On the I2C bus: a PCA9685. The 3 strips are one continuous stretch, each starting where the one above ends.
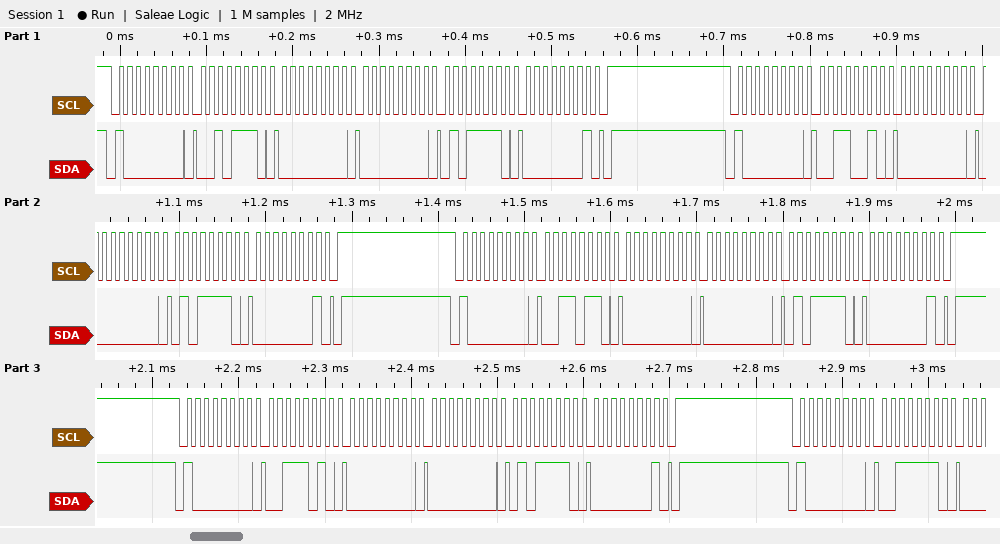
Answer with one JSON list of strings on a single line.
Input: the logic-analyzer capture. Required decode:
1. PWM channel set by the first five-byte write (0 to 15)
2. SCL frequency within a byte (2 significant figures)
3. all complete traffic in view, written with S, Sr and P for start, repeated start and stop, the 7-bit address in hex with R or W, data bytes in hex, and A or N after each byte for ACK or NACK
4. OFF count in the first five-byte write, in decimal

["10", "100 kHz", "S 40W A 2E A 00 A 00 A 5E A 01 A P S 40W A 32 A 00 A 00 A 5E A 01 A P S 40W A 36 A 00 A 00 A 5E A 01 A P S 40W A 3A A 00 A 00 A 5E A 01 A P S 40W A 3E A", "350"]
